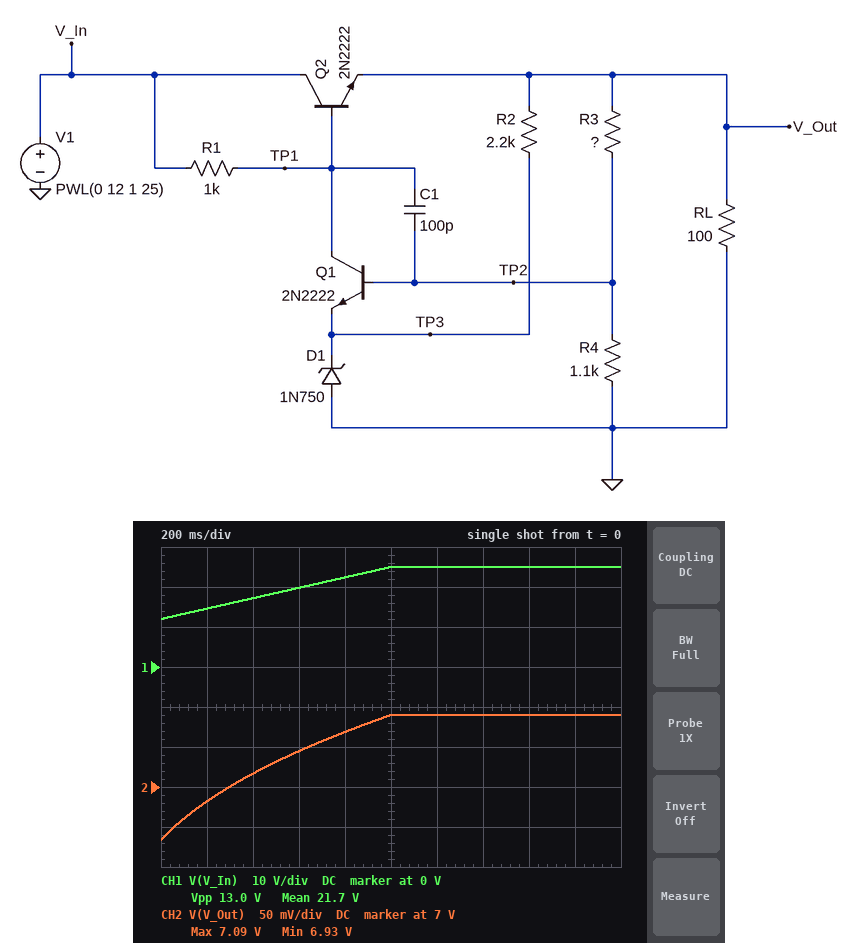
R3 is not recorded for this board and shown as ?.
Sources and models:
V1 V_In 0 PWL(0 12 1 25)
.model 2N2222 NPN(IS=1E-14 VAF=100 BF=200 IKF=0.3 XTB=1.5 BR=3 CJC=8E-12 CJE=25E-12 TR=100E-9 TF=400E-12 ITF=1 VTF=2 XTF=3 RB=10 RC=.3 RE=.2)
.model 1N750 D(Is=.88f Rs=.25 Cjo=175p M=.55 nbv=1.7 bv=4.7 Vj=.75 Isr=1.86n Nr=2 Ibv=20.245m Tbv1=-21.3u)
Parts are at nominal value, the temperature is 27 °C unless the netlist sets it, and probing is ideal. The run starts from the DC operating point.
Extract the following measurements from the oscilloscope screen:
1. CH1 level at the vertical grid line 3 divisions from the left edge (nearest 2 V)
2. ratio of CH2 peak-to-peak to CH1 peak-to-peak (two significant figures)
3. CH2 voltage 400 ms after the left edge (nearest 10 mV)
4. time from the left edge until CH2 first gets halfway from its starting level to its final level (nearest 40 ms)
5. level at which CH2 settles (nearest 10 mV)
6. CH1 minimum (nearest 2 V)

20 V
0.012
7.02 V
360 ms
7.09 V
12 V
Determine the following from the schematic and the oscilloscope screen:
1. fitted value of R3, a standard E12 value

330 Ω
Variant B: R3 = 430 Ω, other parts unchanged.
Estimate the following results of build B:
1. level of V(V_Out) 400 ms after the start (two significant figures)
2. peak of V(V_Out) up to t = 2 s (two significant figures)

7.5 V
7.6 V
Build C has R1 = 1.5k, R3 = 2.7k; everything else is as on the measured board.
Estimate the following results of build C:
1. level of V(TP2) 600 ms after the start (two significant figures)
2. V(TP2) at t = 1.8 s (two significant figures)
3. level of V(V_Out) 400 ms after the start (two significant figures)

4.9 V
5.3 V
15 V
